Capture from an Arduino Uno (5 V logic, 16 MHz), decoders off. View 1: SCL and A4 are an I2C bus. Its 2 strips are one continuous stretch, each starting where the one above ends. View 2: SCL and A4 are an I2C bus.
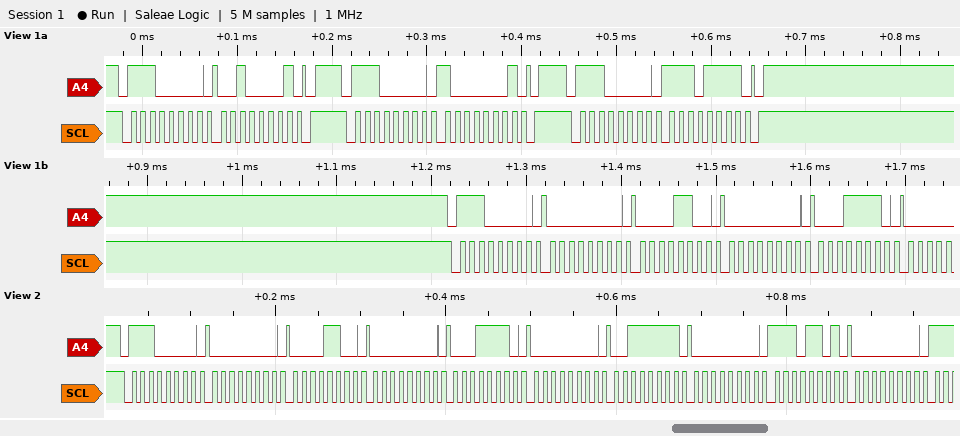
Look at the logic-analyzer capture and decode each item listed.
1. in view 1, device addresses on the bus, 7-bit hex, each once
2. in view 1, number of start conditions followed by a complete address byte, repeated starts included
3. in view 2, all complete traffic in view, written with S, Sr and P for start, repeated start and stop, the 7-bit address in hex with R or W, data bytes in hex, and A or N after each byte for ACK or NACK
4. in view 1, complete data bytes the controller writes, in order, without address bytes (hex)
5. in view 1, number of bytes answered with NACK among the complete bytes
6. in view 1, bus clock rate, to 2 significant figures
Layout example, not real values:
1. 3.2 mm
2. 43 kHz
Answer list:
1. 0x70
2. 4
3. S 70W A 00 A 0C A 00 A 1E A 00 A 3F A 00 A ED A 00 A
4. 21 81 EF 00 0C 00 1E
5. 0
6. 100 kHz
